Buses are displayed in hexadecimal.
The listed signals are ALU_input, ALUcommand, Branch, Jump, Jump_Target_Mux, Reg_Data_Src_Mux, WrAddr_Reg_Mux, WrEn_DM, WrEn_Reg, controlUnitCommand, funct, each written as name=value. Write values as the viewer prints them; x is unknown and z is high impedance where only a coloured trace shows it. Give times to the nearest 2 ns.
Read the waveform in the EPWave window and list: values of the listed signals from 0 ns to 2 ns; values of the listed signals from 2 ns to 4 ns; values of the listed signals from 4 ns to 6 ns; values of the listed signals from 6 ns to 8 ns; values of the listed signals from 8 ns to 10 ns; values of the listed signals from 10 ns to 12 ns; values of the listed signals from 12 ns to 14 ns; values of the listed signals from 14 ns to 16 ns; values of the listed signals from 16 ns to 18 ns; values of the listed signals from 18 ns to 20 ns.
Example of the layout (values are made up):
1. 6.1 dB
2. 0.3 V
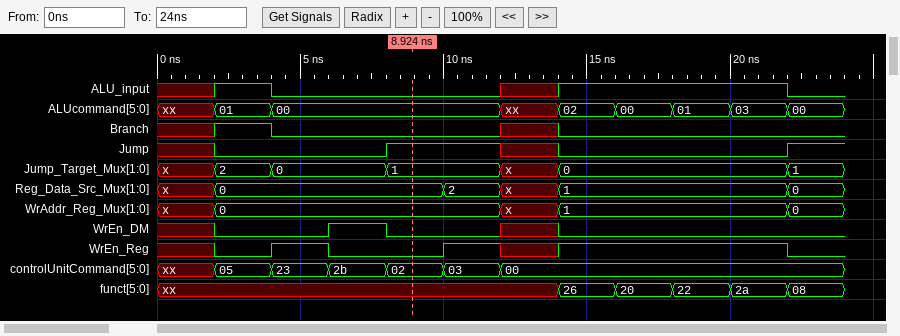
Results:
1. ALU_input=x, ALUcommand=xx, Branch=x, Jump=x, Jump_Target_Mux=x, Reg_Data_Src_Mux=x, WrAddr_Reg_Mux=x, WrEn_DM=x, WrEn_Reg=x, controlUnitCommand=xx, funct=xx
2. ALU_input=1, ALUcommand=01, Branch=1, Jump=0, Jump_Target_Mux=2, Reg_Data_Src_Mux=0, WrAddr_Reg_Mux=0, WrEn_DM=0, WrEn_Reg=0, controlUnitCommand=05, funct=xx
3. ALU_input=0, ALUcommand=00, Branch=0, Jump=0, Jump_Target_Mux=0, Reg_Data_Src_Mux=0, WrAddr_Reg_Mux=0, WrEn_DM=0, WrEn_Reg=1, controlUnitCommand=23, funct=xx
4. ALU_input=0, ALUcommand=00, Branch=0, Jump=0, Jump_Target_Mux=0, Reg_Data_Src_Mux=0, WrAddr_Reg_Mux=0, WrEn_DM=1, WrEn_Reg=0, controlUnitCommand=2b, funct=xx
5. ALU_input=0, ALUcommand=00, Branch=0, Jump=1, Jump_Target_Mux=1, Reg_Data_Src_Mux=0, WrAddr_Reg_Mux=0, WrEn_DM=0, WrEn_Reg=0, controlUnitCommand=02, funct=xx
6. ALU_input=0, ALUcommand=00, Branch=0, Jump=1, Jump_Target_Mux=1, Reg_Data_Src_Mux=2, WrAddr_Reg_Mux=0, WrEn_DM=0, WrEn_Reg=1, controlUnitCommand=03, funct=xx
7. ALU_input=x, ALUcommand=xx, Branch=x, Jump=x, Jump_Target_Mux=x, Reg_Data_Src_Mux=x, WrAddr_Reg_Mux=x, WrEn_DM=x, WrEn_Reg=x, controlUnitCommand=00, funct=xx
8. ALU_input=1, ALUcommand=02, Branch=0, Jump=0, Jump_Target_Mux=0, Reg_Data_Src_Mux=1, WrAddr_Reg_Mux=1, WrEn_DM=0, WrEn_Reg=1, controlUnitCommand=00, funct=26
9. ALU_input=1, ALUcommand=00, Branch=0, Jump=0, Jump_Target_Mux=0, Reg_Data_Src_Mux=1, WrAddr_Reg_Mux=1, WrEn_DM=0, WrEn_Reg=1, controlUnitCommand=00, funct=20
10. ALU_input=1, ALUcommand=01, Branch=0, Jump=0, Jump_Target_Mux=0, Reg_Data_Src_Mux=1, WrAddr_Reg_Mux=1, WrEn_DM=0, WrEn_Reg=1, controlUnitCommand=00, funct=22
